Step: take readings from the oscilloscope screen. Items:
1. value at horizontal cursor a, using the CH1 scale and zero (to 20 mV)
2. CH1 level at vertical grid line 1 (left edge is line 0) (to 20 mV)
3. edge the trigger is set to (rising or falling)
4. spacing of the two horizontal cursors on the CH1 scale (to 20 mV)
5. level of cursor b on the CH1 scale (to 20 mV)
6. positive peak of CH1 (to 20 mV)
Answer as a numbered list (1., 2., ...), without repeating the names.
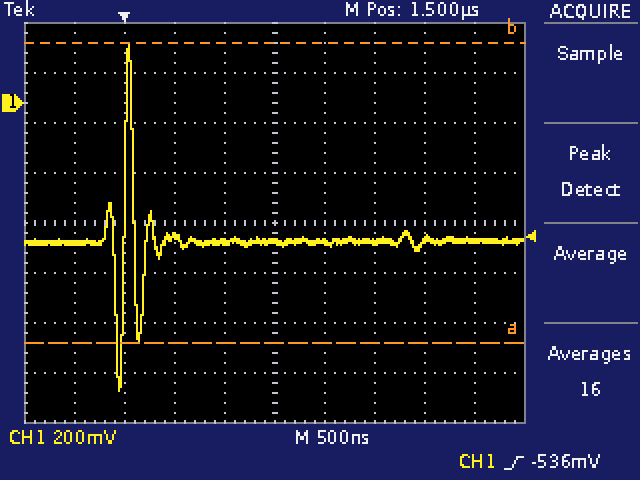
1. -960 mV
2. -560 mV
3. rising
4. 1.20 V
5. 240 mV
6. 240 mV
